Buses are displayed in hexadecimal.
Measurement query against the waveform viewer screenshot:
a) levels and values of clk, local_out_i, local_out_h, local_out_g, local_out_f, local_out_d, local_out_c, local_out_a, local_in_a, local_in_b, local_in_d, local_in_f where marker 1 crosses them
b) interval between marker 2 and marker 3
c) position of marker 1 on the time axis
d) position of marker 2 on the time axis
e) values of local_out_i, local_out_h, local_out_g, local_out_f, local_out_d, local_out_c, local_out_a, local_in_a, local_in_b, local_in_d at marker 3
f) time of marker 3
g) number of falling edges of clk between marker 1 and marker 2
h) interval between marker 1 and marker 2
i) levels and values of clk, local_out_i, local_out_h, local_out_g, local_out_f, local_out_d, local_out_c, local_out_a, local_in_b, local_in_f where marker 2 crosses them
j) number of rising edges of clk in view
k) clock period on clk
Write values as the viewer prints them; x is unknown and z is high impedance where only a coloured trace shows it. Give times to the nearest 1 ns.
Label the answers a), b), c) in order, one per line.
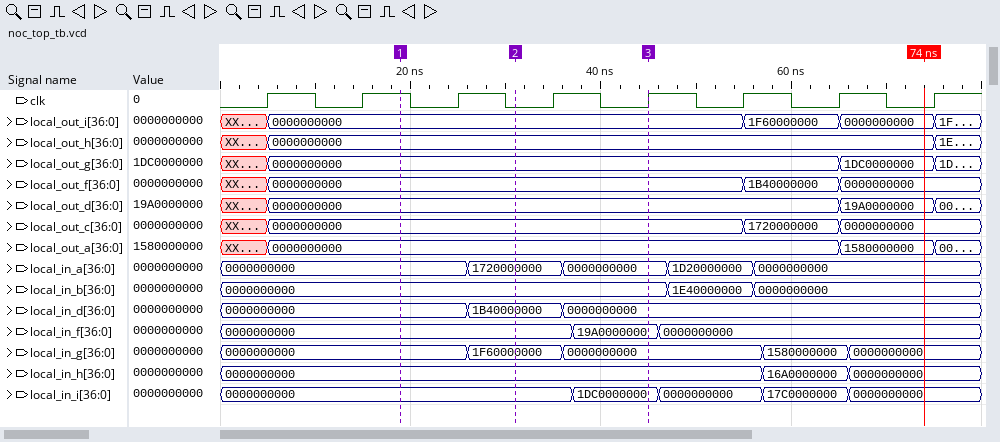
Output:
a) clk=1, local_out_i=0000000000, local_out_h=0000000000, local_out_g=0000000000, local_out_f=0000000000, local_out_d=0000000000, local_out_c=0000000000, local_out_a=0000000000, local_in_a=0000000000, local_in_b=0000000000, local_in_d=0000000000, local_in_f=0000000000
b) 14 ns
c) 19 ns
d) 31 ns
e) local_out_i=0000000000, local_out_h=0000000000, local_out_g=0000000000, local_out_f=0000000000, local_out_d=0000000000, local_out_c=0000000000, local_out_a=0000000000, local_in_a=0000000000, local_in_b=0000000000, local_in_d=0000000000
f) 45 ns
g) 2
h) 12 ns
i) clk=0, local_out_i=0000000000, local_out_h=0000000000, local_out_g=0000000000, local_out_f=0000000000, local_out_d=0000000000, local_out_c=0000000000, local_out_a=0000000000, local_in_b=0000000000, local_in_f=0000000000
j) 8
k) 10 ns
